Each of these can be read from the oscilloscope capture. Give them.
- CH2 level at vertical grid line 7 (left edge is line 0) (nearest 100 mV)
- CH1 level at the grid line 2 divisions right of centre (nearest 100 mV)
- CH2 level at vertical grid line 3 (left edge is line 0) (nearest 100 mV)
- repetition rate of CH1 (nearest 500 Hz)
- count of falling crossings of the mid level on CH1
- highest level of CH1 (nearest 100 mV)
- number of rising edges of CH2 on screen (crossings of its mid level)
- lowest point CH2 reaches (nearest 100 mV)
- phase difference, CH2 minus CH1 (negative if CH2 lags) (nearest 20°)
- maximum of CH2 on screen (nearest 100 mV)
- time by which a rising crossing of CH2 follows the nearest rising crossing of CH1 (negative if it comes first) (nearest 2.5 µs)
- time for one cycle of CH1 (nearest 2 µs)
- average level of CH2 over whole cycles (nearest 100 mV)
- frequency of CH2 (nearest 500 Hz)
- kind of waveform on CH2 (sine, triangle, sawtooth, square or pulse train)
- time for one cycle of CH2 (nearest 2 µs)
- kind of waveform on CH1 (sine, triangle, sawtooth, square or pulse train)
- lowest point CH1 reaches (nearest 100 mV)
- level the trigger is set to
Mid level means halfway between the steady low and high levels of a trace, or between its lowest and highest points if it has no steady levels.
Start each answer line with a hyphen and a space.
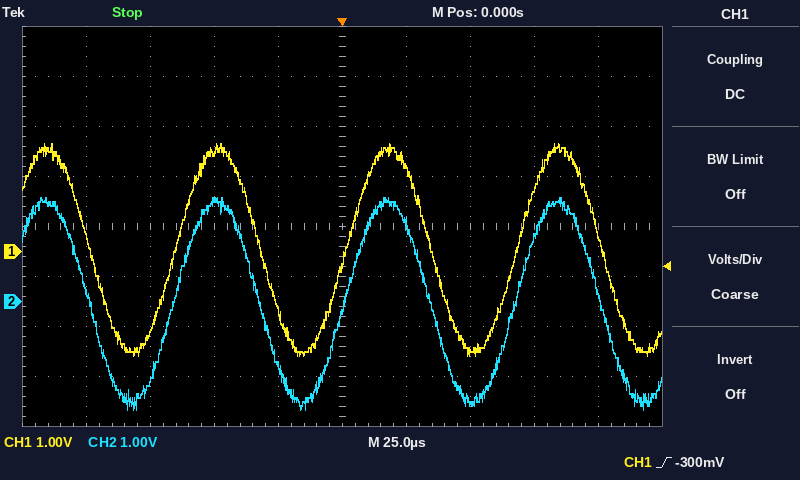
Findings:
- -2.0 V
- -2.0 V
- 2.0 V
- 15.0 kHz
- 4
- 2.2 V
- 3
- -2.2 V
- 0°
- 2.1 V
- 0.0 µs
- 66 µs
- 0.0 V
- 15.0 kHz
- sine
- 66 µs
- sine
- -2.1 V
- -300 mV
